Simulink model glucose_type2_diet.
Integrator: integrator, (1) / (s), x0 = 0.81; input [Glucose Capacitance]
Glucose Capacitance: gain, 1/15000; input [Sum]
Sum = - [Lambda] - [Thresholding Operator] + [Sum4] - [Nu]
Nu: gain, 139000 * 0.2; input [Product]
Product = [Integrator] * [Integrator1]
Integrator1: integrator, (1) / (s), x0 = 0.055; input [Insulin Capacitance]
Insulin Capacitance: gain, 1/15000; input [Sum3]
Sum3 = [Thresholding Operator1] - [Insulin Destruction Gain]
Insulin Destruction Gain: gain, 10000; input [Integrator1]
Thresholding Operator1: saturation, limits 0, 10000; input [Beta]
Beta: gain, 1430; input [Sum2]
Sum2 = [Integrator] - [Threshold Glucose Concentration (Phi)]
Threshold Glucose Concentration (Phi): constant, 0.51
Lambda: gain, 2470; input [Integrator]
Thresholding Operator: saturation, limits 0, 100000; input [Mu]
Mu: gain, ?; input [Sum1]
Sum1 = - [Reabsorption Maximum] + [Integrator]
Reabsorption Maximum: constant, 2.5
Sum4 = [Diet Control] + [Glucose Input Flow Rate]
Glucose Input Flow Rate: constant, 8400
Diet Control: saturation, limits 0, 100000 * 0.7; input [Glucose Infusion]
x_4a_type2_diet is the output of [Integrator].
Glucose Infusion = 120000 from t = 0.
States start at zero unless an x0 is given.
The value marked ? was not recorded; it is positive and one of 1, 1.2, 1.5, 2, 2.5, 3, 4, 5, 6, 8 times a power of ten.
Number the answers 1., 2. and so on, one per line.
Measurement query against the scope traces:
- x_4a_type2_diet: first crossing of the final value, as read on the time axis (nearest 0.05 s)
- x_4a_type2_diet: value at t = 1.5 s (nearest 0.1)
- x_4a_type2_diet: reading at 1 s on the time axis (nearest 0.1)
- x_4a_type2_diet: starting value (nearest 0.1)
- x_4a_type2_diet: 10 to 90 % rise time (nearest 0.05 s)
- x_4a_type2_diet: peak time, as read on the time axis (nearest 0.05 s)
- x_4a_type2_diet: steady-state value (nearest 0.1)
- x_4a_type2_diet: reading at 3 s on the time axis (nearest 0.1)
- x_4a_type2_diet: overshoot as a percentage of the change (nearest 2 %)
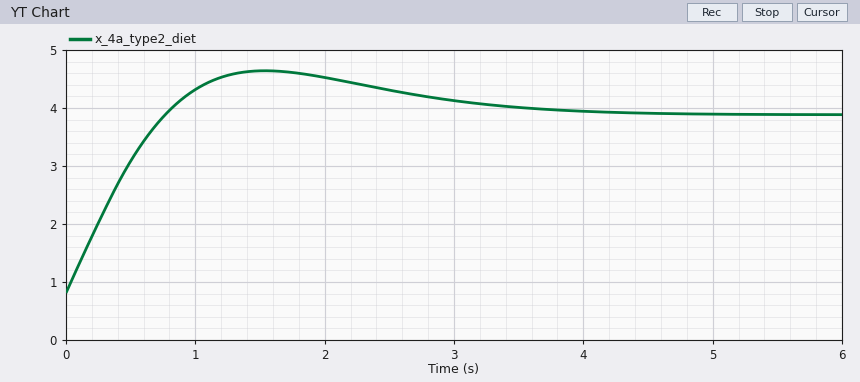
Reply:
1. 0.75 s
2. 4.6
3. 4.3
4. 0.8
5. 0.60 s
6. 1.55 s
7. 3.9
8. 4.1
9. 24 %
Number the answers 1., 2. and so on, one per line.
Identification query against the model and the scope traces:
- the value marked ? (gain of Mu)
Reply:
1. 12000
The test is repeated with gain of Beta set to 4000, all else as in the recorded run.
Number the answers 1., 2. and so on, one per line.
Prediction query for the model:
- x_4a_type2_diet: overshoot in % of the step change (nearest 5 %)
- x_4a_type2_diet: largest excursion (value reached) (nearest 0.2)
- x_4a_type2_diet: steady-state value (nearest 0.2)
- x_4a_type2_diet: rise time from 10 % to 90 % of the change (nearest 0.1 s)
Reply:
1. 55 %
2. 3.8
3. 2.8
4. 0.3 s
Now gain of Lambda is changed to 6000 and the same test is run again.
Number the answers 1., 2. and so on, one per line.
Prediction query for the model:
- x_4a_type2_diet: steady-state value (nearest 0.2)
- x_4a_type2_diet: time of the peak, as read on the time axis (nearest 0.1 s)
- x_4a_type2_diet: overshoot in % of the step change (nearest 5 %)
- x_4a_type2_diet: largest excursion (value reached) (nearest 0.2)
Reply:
1. 3.6
2. 1.5 s
3. 20 %
4. 4.2
